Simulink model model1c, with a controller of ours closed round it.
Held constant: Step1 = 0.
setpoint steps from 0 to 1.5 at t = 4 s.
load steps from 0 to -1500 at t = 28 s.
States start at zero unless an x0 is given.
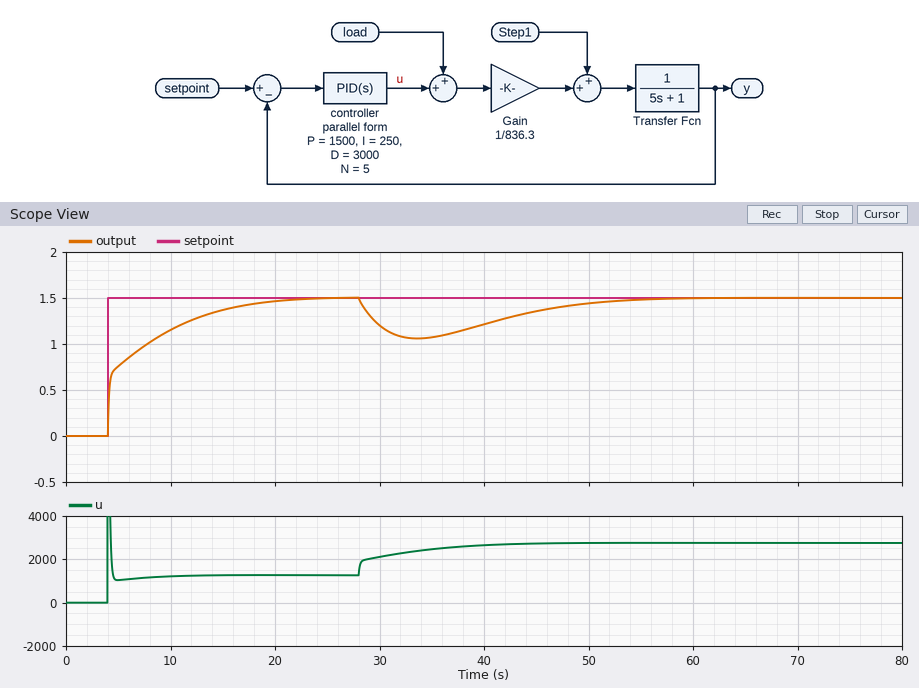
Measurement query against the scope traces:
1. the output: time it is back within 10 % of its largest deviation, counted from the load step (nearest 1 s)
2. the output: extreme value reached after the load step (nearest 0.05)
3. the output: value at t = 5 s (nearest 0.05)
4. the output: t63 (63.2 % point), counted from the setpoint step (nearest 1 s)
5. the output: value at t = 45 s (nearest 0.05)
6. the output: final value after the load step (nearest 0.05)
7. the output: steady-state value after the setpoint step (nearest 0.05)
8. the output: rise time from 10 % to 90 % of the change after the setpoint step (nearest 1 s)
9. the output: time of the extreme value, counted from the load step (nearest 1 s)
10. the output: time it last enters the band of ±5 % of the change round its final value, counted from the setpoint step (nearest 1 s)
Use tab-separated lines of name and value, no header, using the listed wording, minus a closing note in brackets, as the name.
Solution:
the output: time it is back within 10 % of its largest deviation, counted from the load step	23 s
the output: extreme value reached after the load step	1.05
the output: value at t = 5 s	0.75
the output: t63 (63.2 % point), counted from the setpoint step	3 s
the output: value at t = 45 s	1.35
the output: final value after the load step	1.50
the output: steady-state value after the setpoint step	1.50
the output: rise time from 10 % to 90 % of the change after the setpoint step	10 s
the output: time of the extreme value, counted from the load step	6 s
the output: time it last enters the band of ±5 % of the change round its final value, counted from the setpoint step	13 s
